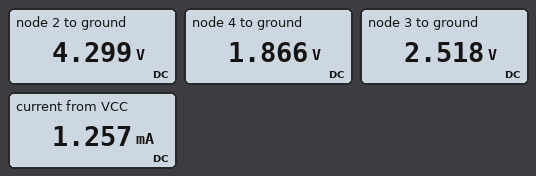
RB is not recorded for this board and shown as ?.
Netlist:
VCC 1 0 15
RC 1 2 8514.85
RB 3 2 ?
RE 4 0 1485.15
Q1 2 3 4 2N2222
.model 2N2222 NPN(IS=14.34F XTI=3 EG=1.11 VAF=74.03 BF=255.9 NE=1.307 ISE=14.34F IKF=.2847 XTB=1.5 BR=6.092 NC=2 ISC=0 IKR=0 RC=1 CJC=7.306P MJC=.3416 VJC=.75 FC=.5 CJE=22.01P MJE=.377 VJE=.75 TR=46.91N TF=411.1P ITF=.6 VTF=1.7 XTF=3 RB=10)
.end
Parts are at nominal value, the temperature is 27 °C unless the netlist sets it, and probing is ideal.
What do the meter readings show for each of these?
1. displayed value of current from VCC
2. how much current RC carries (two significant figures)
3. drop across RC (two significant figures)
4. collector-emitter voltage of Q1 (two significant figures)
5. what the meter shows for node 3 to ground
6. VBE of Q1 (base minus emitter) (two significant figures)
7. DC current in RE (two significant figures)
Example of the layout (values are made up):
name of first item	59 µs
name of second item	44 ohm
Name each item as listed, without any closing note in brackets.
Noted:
displayed value of current from VCC	1.257 mA
how much current RC carries	1.3 mA
drop across RC	11 V
collector-emitter voltage of Q1	2.4 V
what the meter shows for node 3 to ground	2.518 V
VBE of Q1 (base minus emitter)	650 mV
DC current in RE	1.3 mA
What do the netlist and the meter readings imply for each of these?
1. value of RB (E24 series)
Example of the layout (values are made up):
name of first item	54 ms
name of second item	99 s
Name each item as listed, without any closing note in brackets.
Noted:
value of RB	220 kΩ
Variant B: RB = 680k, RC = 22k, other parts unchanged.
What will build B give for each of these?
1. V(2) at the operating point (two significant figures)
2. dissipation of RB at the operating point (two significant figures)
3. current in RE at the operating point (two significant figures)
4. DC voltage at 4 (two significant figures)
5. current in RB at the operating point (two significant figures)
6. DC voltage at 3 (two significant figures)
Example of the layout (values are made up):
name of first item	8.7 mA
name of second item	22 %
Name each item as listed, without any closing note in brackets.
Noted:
V(2) at the operating point	3.8 V
dissipation of RB at the operating point	8.6 µW
current in RE at the operating point	510 µA
DC voltage at 4	760 mV
current in RB at the operating point	3.6 µA
DC voltage at 3	1.4 V
